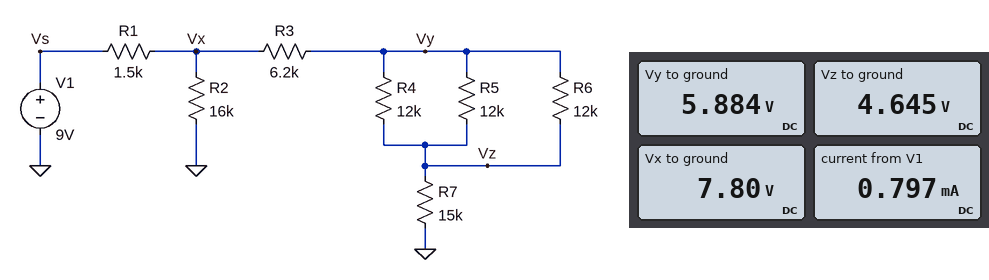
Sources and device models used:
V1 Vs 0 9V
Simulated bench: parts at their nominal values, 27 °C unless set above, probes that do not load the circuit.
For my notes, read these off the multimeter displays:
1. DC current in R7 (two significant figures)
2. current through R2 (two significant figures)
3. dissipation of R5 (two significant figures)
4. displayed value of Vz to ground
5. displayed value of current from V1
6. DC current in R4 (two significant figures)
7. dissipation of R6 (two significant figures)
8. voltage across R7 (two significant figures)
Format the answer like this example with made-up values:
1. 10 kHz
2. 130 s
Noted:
1. 310 µA
2. 490 µA
3. 130 µW
4. 4.645 V
5. 0.797 mA
6. 100 µA
7. 130 µW
8. 4.6 V
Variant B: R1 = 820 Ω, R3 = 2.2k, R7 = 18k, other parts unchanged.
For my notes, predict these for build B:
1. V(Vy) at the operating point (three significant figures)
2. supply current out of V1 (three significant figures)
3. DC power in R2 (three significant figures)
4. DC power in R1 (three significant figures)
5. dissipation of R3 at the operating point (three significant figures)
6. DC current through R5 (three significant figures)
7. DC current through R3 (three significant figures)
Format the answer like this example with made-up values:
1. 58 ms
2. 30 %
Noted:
1. 7.54 V
2. 861 µA
3. 4.30 mW
4. 608 µW
5. 258 µW
6. 114 µA
7. 343 µA
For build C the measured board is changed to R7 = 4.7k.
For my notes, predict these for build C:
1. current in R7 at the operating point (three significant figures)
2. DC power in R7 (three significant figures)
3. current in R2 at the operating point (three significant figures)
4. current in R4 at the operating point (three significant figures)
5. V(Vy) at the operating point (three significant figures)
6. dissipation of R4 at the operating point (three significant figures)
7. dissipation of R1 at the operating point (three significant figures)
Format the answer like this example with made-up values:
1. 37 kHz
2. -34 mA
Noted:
1. 506 µA
2. 1.20 mW
3. 471 µA
4. 169 µA
5. 4.40 V
6. 341 µW
7. 1.43 mW
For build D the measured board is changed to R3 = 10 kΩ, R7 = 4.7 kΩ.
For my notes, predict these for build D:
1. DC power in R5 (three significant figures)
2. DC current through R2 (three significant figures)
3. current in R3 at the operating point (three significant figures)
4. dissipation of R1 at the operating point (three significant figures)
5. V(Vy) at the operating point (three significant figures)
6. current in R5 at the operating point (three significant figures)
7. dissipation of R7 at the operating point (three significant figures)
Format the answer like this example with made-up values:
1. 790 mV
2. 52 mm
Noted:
1. 224 µW
2. 479 µA
3. 410 µA
4. 1.19 mW
5. 3.57 V
6. 137 µA
7. 790 µW
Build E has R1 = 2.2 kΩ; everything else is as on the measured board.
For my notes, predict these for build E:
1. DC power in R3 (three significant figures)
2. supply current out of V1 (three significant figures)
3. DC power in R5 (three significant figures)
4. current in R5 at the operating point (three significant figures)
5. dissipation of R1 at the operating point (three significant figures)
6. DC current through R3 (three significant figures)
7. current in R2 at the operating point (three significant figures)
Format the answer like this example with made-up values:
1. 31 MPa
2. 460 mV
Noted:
1. 527 µW
2. 751 µA
3. 113 µW
4. 97.2 µA
5. 1.24 mW
6. 292 µA
7. 459 µA
